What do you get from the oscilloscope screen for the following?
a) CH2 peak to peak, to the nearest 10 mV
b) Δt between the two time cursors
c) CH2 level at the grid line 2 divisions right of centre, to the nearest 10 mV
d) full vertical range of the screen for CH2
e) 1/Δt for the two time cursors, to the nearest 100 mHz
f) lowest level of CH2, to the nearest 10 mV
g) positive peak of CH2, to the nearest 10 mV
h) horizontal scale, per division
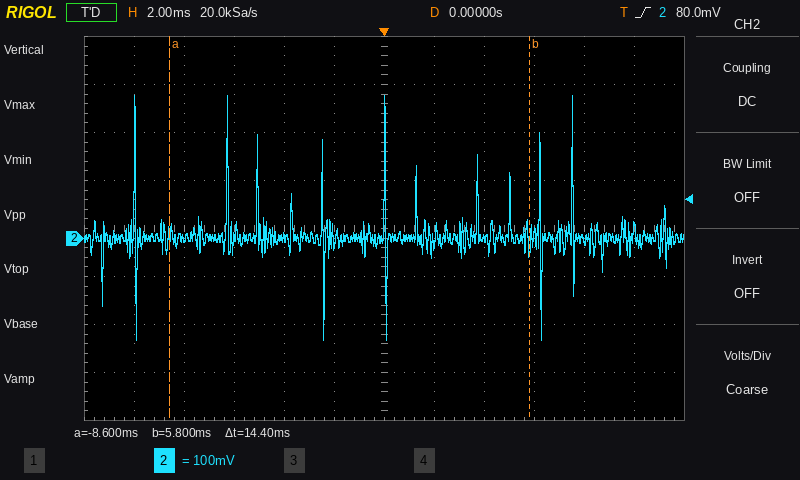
510 mV
14.4 ms
0 mV
800 mV
69.4 Hz
-210 mV
300 mV
2 ms
